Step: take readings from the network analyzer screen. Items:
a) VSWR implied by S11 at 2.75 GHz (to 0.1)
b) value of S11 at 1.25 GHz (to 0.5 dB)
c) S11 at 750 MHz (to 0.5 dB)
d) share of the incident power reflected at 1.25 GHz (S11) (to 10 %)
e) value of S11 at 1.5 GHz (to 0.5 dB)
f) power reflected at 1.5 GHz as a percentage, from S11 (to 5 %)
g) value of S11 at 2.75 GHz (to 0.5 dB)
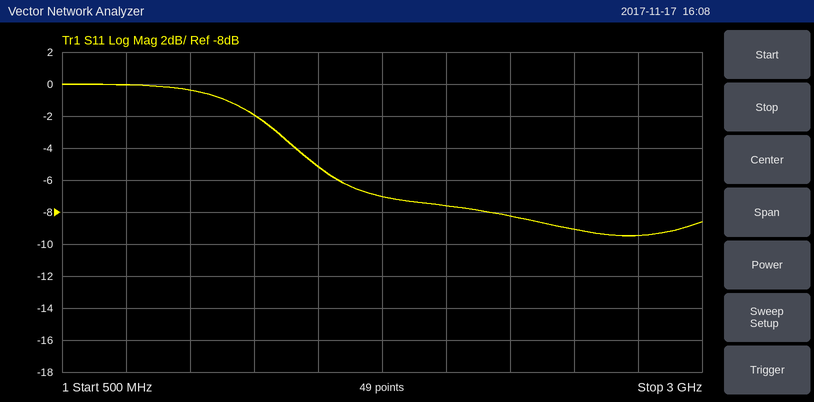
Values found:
2.0
-2.0 dB
0.0 dB
60 %
-5.0 dB
30 %
-9.5 dB
